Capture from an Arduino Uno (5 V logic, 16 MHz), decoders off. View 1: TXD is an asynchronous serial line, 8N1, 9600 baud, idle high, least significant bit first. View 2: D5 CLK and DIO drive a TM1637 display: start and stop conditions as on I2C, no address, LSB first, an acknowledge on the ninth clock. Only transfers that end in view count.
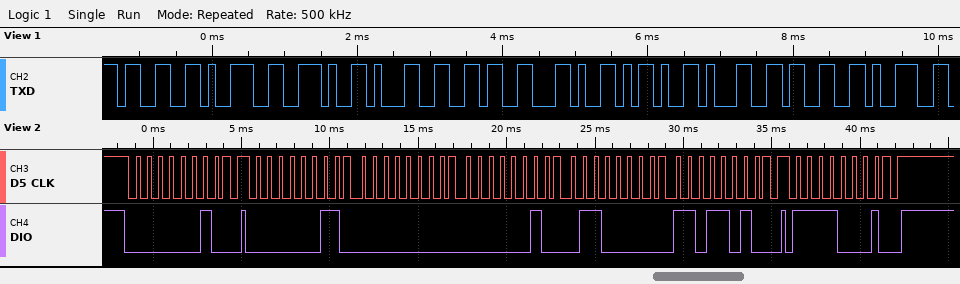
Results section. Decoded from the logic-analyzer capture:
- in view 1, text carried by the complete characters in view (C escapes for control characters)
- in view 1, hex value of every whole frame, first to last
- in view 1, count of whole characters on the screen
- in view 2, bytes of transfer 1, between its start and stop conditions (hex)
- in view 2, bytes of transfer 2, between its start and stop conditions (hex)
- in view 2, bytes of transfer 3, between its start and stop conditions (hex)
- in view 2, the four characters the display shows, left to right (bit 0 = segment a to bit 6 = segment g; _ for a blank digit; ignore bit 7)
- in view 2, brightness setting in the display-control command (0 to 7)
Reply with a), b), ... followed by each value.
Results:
a) "39.16,-139"
b) 33 39 2E 31 36 2C 2D 31 33 39
c) 10
d) 40
e) C0 00 40 06 5B
f) 8F
g) _-12
h) 7
